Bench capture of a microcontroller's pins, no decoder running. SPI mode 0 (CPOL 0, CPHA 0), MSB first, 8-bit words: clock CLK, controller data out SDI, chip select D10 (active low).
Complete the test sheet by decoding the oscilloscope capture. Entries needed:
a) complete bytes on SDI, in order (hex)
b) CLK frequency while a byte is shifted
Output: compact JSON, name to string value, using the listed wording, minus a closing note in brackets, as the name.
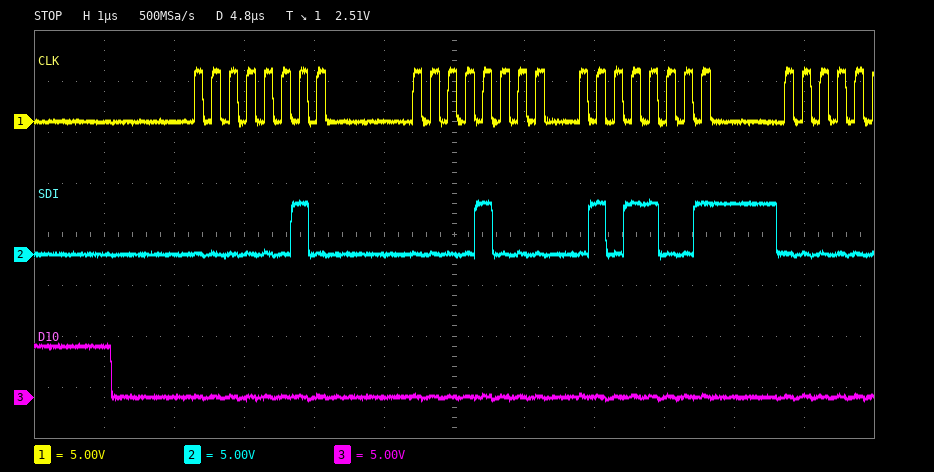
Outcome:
{"complete bytes on SDI, in order": "02 08 59", "CLK frequency while a byte is shifted": "4 MHz"}
